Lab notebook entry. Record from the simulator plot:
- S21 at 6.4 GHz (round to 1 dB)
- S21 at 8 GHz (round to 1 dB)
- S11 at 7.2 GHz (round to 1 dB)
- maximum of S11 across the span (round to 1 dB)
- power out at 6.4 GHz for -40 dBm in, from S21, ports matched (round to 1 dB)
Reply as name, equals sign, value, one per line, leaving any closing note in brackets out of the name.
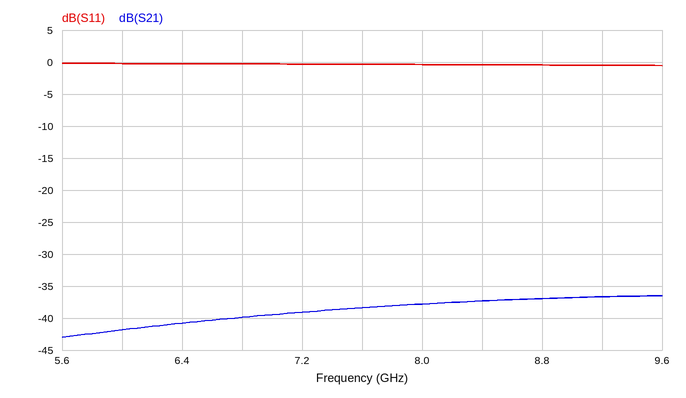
S21 at 6.4 GHz = -41 dB
S21 at 8 GHz = -38 dB
S11 at 7.2 GHz = 0 dB
maximum of S11 across the span = 0 dB
power out at 6.4 GHz for -40 dBm in, from S21, ports matched = -81 dBm
